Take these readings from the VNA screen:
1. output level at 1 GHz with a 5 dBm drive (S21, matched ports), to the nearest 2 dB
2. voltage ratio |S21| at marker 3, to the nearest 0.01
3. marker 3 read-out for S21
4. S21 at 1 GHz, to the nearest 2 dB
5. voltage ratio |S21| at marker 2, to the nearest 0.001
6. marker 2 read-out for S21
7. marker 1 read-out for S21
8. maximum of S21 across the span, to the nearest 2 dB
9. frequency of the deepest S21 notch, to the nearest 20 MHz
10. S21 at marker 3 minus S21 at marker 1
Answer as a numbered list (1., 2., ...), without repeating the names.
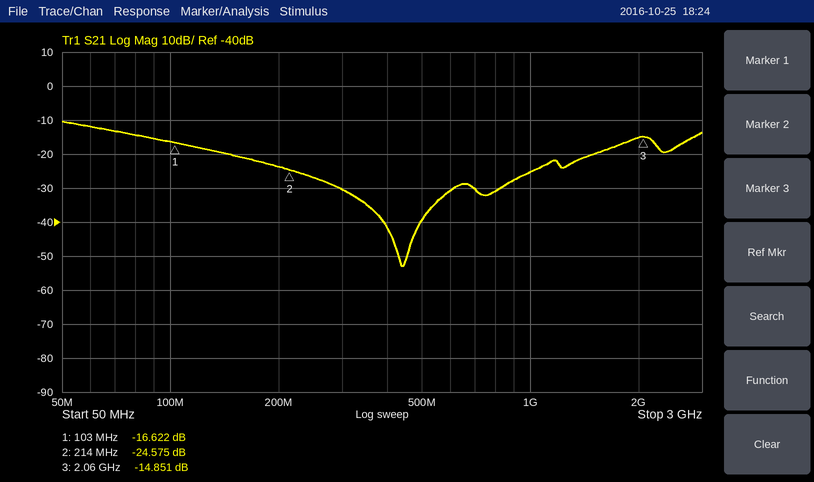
1. -20 dBm
2. 0.18
3. -14.851 dB
4. -26 dB
5. 0.059
6. -24.575 dB
7. -16.622 dB
8. -10 dB
9. 440 MHz
10. 1.771 dB
